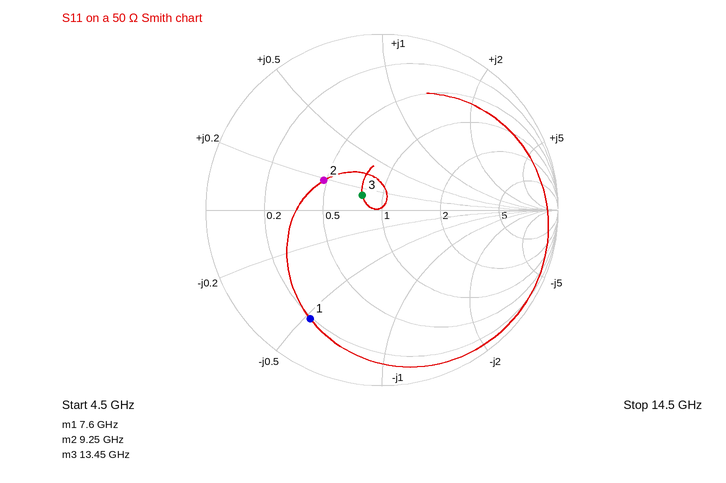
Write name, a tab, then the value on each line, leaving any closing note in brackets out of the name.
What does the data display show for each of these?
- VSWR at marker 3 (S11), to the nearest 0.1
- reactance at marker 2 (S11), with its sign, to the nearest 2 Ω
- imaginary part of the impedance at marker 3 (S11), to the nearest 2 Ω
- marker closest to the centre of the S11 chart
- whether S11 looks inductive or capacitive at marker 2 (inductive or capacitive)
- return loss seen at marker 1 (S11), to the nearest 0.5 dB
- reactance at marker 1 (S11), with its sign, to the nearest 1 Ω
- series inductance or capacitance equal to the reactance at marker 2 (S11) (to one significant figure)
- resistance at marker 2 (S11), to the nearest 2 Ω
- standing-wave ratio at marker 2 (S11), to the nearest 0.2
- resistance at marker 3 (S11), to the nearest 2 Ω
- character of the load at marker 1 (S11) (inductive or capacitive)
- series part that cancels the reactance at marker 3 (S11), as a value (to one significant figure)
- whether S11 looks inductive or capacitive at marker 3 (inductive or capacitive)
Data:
VSWR at marker 3 (S11), to the nearest 0.1	1.3
reactance at marker 2 (S11), with its sign, to the nearest 2 Ω	+10 Ω
imaginary part of the impedance at marker 3 (S11), to the nearest 2 Ω	+6 Ω
marker closest to the centre of the S11 chart	marker 3
whether S11 looks inductive or capacitive at marker 2	inductive
return loss seen at marker 1 (S11), to the nearest 0.5 dB	2.5 dB
reactance at marker 1 (S11), with its sign, to the nearest 1 Ω	-26 Ω
series inductance or capacitance equal to the reactance at marker 2 (S11)	200 pH
resistance at marker 2 (S11), to the nearest 2 Ω	24 Ω
standing-wave ratio at marker 2 (S11), to the nearest 0.2	2.2
resistance at marker 3 (S11), to the nearest 2 Ω	40 Ω
character of the load at marker 1 (S11)	capacitive
series part that cancels the reactance at marker 3 (S11), as a value	2 pF
whether S11 looks inductive or capacitive at marker 3	inductive
